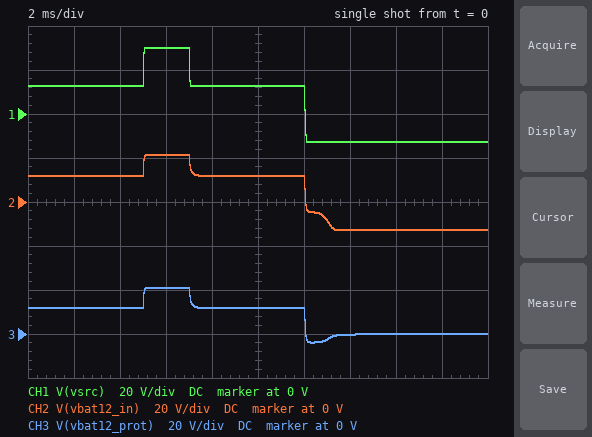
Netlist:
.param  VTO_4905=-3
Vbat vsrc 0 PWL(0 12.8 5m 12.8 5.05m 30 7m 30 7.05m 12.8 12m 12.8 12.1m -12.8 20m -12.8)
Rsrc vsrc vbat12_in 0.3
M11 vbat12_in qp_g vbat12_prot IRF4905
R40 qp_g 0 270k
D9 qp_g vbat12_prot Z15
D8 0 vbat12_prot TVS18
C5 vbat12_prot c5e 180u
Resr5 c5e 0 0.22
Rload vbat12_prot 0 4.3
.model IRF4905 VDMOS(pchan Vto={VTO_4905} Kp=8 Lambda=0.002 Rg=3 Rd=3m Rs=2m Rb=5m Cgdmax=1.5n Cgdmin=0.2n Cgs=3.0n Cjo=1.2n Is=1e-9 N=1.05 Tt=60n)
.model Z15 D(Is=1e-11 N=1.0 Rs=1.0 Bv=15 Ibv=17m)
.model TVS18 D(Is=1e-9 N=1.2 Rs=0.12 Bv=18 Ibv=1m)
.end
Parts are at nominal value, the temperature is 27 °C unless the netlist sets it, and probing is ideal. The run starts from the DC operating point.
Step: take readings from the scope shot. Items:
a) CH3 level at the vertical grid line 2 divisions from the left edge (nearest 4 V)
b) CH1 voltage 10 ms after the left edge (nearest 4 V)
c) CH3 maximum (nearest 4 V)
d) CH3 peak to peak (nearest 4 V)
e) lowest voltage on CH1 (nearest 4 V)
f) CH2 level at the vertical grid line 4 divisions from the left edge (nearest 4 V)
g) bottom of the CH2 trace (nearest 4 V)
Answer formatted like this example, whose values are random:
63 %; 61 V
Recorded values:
12 V; 12 V; 20 V; 24 V; -12 V; 12 V; -12 V
